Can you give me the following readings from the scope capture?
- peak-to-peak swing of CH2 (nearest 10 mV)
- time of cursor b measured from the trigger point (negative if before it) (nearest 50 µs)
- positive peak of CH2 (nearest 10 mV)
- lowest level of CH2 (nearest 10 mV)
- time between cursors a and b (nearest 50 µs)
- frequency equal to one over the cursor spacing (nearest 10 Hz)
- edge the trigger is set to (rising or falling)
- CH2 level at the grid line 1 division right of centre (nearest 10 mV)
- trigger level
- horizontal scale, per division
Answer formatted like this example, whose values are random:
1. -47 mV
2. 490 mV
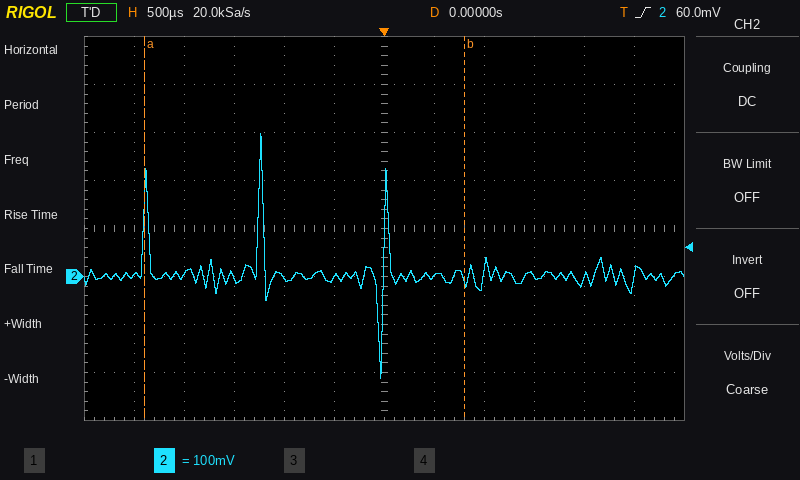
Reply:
1. 510 mV
2. +800 µs
3. 300 mV
4. -210 mV
5. 3.20 ms
6. 310 Hz
7. rising
8. 0 mV
9. 60.0 mV
10. 500 µs
